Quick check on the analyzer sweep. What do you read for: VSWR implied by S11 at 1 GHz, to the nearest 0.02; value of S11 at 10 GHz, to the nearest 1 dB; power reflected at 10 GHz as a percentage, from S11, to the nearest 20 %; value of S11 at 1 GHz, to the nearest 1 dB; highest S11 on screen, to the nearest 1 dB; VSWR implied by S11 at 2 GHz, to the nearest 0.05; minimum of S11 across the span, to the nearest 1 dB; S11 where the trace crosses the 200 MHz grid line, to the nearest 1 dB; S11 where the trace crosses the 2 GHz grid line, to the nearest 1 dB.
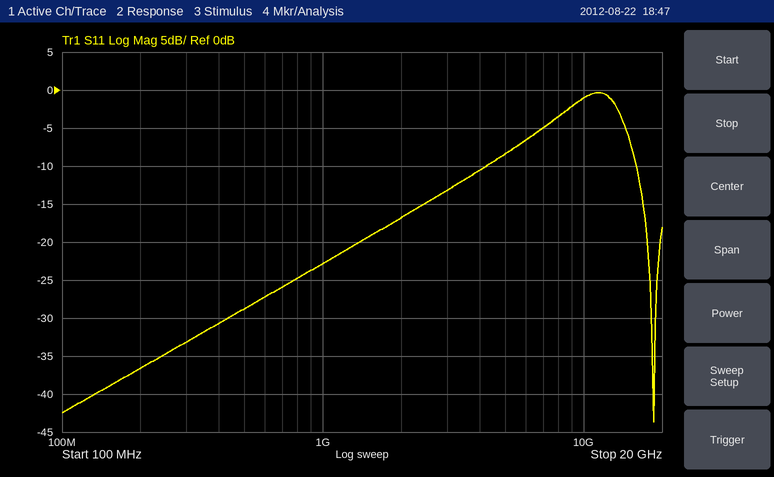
1.16
-1 dB
80 %
-23 dB
0 dB
1.35
-44 dB
-37 dB
-17 dB
